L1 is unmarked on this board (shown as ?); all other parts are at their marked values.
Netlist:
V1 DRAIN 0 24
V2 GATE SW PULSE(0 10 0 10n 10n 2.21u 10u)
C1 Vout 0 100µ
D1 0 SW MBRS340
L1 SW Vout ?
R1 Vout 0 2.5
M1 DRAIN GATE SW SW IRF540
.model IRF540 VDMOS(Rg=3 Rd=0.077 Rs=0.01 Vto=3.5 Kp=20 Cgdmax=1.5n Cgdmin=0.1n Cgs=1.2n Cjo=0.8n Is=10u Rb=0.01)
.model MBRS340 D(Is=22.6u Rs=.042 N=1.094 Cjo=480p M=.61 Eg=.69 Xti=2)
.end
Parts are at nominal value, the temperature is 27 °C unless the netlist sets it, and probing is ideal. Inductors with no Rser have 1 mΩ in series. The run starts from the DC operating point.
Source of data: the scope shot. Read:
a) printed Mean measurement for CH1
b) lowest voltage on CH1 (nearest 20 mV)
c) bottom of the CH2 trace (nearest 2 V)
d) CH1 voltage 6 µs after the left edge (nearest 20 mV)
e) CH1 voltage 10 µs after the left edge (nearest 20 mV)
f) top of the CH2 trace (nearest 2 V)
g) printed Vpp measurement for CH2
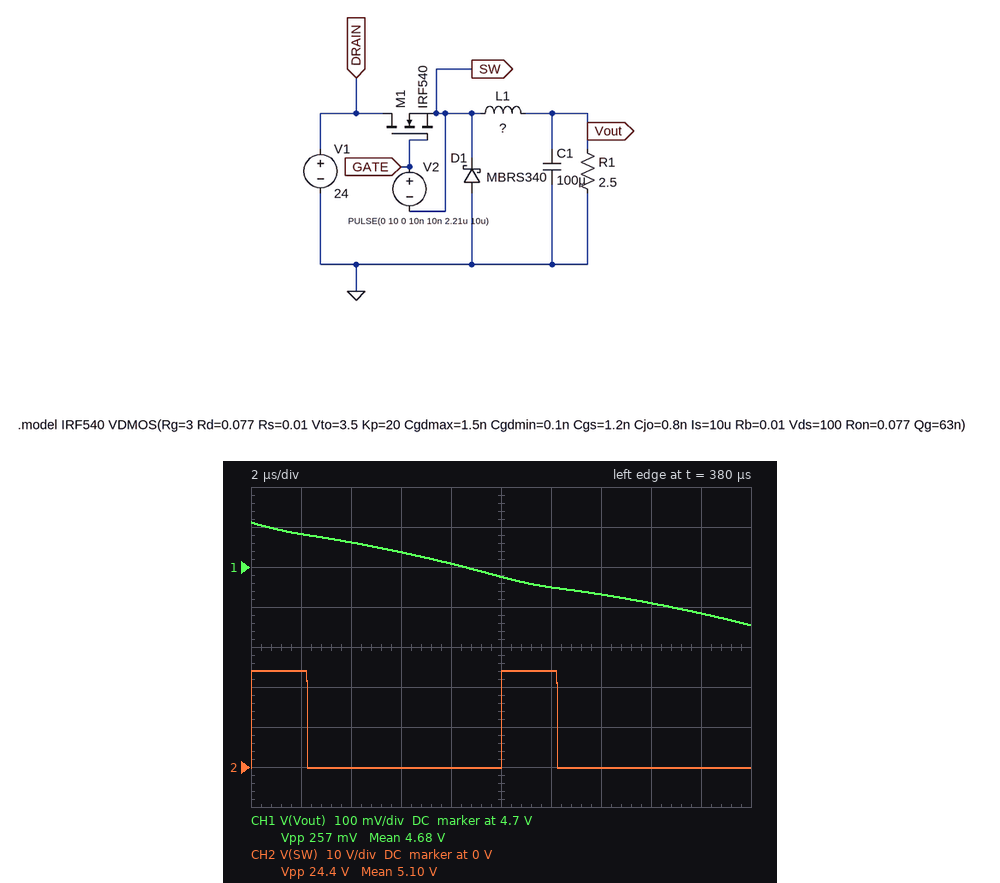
4.68 V
4.56 V
0 V
4.74 V
4.68 V
24 V
24.4 V
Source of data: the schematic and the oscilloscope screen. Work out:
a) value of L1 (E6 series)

47 µH
